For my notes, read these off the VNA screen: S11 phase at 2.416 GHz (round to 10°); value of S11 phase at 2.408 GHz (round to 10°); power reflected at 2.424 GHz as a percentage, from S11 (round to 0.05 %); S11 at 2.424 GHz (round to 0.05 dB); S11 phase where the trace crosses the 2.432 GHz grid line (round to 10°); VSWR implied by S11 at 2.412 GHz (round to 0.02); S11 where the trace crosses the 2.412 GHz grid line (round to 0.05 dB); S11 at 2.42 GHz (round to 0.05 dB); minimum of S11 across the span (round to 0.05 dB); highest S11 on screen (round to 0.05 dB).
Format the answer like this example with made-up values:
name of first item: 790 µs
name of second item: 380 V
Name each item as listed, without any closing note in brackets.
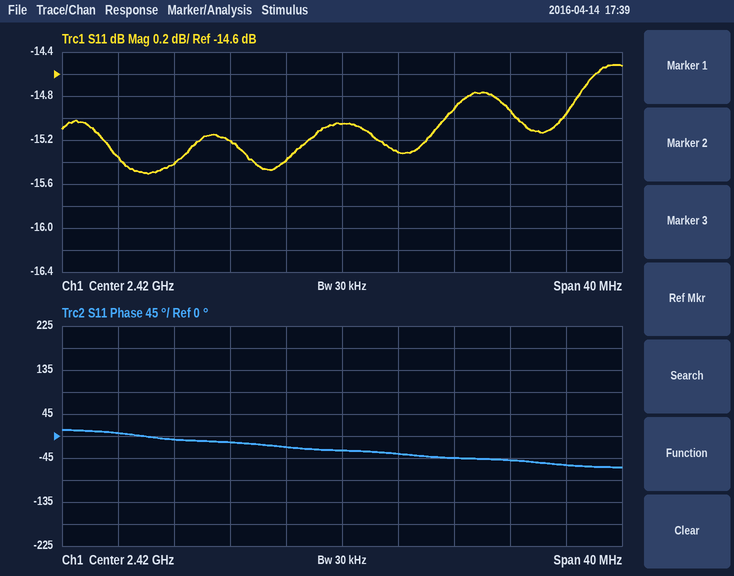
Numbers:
S11 phase at 2.416 GHz: -20°
value of S11 phase at 2.408 GHz: -10°
power reflected at 2.424 GHz as a percentage, from S11: 2.95 %
S11 at 2.424 GHz: -15.30 dB
S11 phase where the trace crosses the 2.432 GHz grid line: -50°
VSWR implied by S11 at 2.412 GHz: 1.42
S11 where the trace crosses the 2.412 GHz grid line: -15.20 dB
S11 at 2.42 GHz: -15.05 dB
minimum of S11 across the span: -15.50 dB
highest S11 on screen: -14.50 dB
